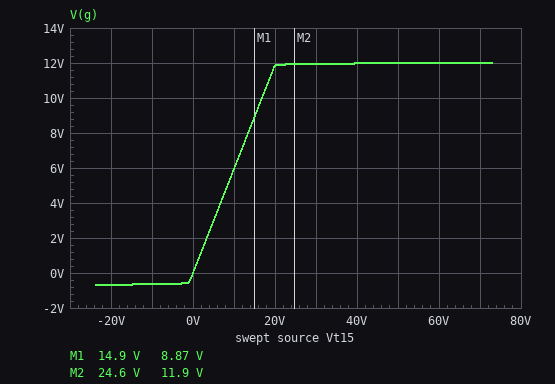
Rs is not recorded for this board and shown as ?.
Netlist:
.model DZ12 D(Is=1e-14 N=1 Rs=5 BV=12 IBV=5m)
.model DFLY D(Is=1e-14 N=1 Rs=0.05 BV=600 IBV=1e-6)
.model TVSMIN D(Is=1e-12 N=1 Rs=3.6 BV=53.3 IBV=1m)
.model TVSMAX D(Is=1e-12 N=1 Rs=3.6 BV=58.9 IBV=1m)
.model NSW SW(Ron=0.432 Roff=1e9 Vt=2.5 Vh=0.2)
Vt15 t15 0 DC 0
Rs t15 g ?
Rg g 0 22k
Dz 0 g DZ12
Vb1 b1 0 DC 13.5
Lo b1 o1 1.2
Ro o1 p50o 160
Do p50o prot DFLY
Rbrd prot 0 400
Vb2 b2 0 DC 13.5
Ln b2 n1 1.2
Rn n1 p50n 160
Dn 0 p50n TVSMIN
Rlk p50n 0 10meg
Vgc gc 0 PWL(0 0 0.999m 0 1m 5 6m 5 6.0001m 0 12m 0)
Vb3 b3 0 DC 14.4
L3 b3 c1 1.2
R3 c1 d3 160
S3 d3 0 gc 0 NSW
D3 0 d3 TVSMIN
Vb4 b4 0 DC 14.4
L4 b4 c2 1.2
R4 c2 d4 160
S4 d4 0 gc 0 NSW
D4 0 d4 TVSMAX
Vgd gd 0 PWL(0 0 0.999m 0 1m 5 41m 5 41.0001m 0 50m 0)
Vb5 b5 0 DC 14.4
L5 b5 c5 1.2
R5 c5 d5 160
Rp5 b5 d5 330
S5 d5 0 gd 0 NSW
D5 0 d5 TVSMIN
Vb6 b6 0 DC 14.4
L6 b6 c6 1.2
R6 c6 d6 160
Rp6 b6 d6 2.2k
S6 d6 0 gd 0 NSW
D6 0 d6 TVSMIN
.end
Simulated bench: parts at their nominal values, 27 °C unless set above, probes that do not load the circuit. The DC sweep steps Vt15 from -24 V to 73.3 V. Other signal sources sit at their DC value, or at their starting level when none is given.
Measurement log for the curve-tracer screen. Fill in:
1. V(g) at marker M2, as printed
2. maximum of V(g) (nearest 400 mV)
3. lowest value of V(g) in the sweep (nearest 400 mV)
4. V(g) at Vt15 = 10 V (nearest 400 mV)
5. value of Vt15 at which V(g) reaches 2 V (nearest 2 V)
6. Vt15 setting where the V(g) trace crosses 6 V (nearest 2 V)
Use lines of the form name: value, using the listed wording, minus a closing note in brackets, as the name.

V(g) at marker M2, as printed: 11.9 V
maximum of V(g): 12.0 V
lowest value of V(g) in the sweep: -800 mV
V(g) at Vt15 = 10 V: 6.0 V
value of Vt15 at which V(g) reaches 2 V: 4 V
Vt15 setting where the V(g) trace crosses 6 V: 10 V
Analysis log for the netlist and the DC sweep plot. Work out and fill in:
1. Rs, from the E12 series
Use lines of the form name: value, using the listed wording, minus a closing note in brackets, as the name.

Rs, from the E12 series: 15 kΩ
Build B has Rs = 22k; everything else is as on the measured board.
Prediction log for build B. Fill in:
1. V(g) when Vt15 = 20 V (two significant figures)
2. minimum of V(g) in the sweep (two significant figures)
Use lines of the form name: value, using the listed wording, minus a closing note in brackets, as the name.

V(g) when Vt15 = 20 V: 10 V
minimum of V(g) in the sweep: -660 mV
